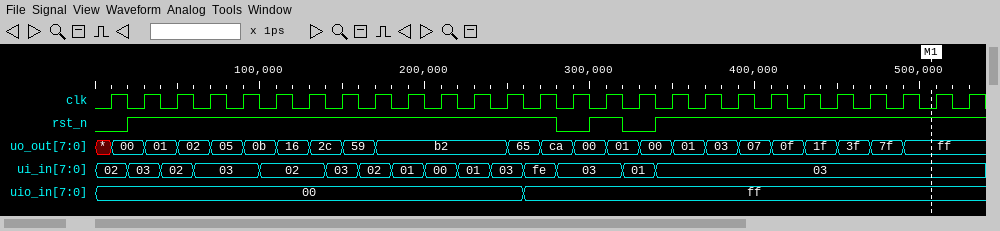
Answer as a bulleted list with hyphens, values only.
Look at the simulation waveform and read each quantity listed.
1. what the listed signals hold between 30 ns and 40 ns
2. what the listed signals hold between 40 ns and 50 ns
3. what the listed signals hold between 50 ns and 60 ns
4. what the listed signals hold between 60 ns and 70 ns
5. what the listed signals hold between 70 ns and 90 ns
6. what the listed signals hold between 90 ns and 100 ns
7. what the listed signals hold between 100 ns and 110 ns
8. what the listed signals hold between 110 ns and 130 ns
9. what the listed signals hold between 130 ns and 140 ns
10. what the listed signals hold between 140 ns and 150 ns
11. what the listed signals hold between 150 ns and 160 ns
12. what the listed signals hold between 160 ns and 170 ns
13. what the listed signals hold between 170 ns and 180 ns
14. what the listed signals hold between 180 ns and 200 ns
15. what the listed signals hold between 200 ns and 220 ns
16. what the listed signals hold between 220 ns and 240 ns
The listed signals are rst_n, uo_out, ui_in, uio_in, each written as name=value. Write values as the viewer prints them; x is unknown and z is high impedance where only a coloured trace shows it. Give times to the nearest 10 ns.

- rst_n=1, uo_out=01, ui_in=03, uio_in=00
- rst_n=1, uo_out=01, ui_in=02, uio_in=00
- rst_n=1, uo_out=02, ui_in=02, uio_in=00
- rst_n=1, uo_out=02, ui_in=03, uio_in=00
- rst_n=1, uo_out=05, ui_in=03, uio_in=00
- rst_n=1, uo_out=0b, ui_in=03, uio_in=00
- rst_n=1, uo_out=0b, ui_in=02, uio_in=00
- rst_n=1, uo_out=16, ui_in=02, uio_in=00
- rst_n=1, uo_out=2c, ui_in=02, uio_in=00
- rst_n=1, uo_out=2c, ui_in=03, uio_in=00
- rst_n=1, uo_out=59, ui_in=03, uio_in=00
- rst_n=1, uo_out=59, ui_in=02, uio_in=00
- rst_n=1, uo_out=b2, ui_in=02, uio_in=00
- rst_n=1, uo_out=b2, ui_in=01, uio_in=00
- rst_n=1, uo_out=b2, ui_in=00, uio_in=00
- rst_n=1, uo_out=b2, ui_in=01, uio_in=00
